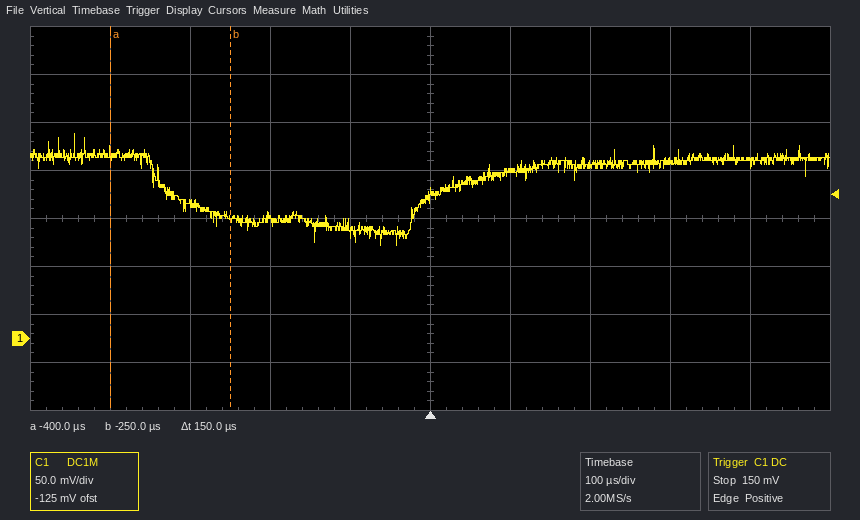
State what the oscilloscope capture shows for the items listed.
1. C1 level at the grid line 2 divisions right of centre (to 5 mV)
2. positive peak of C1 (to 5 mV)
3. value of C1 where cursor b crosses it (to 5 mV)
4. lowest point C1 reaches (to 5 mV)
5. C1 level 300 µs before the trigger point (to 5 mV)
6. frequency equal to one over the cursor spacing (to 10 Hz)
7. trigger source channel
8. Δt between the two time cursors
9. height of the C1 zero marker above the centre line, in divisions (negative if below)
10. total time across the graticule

180 mV
215 mV
125 mV
95 mV
140 mV
6.67 kHz
C1
150 µs
-2.5 div
1 ms
